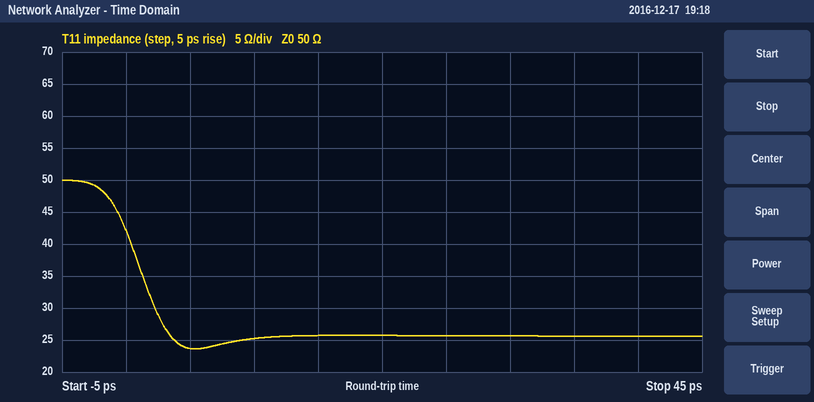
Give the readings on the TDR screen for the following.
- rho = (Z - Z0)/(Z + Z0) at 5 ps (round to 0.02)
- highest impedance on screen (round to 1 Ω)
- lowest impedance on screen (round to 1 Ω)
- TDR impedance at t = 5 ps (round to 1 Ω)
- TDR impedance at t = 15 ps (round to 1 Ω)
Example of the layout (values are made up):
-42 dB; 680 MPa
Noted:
-0.36; 50 Ω; 24 Ω; 24 Ω; 26 Ω
